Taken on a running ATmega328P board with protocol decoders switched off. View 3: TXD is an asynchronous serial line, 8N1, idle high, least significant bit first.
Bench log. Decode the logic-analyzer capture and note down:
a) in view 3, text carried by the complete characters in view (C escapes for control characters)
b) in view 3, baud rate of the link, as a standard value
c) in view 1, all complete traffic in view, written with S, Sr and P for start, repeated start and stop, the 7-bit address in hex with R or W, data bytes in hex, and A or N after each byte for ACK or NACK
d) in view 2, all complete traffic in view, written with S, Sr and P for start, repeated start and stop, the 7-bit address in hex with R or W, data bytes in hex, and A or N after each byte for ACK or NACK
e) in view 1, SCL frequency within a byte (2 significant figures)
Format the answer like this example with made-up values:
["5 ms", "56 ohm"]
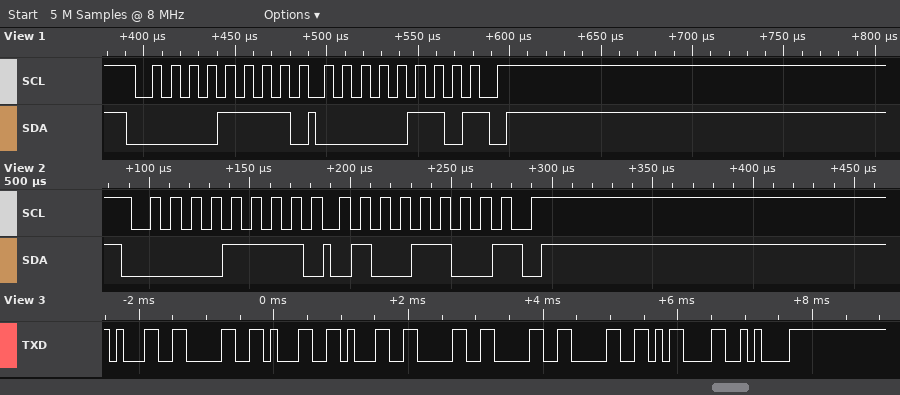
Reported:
["\"1011000\\r\\n\"", "9600 baud", "S 07R A 06 N P", "S 07R A 4C N P", "100 kHz"]
